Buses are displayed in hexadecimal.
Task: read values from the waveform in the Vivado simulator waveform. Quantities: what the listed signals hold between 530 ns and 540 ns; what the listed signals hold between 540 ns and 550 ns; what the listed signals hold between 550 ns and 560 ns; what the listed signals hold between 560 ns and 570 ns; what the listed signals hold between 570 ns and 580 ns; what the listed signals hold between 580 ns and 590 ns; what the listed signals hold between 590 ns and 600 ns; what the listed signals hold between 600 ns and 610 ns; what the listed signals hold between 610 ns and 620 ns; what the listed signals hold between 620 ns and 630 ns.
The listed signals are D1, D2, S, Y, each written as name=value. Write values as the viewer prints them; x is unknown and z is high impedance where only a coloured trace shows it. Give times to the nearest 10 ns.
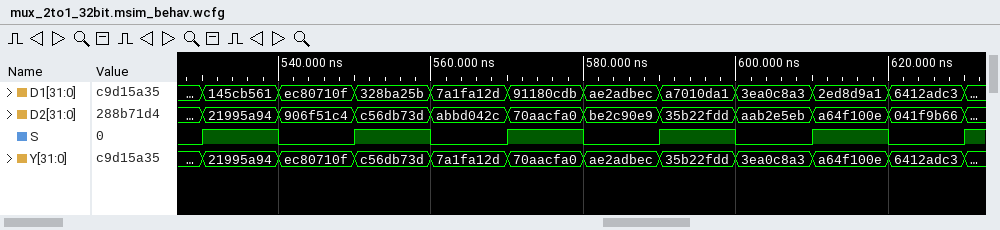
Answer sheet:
D1=145cb561, D2=21995a94, S=1, Y=21995a94
D1=ec80710f, D2=906f51c4, S=0, Y=ec80710f
D1=328ba25b, D2=c56db73d, S=1, Y=c56db73d
D1=7a1fa12d, D2=abbd042c, S=0, Y=7a1fa12d
D1=91180cdb, D2=70aacfa0, S=1, Y=70aacfa0
D1=ae2adbec, D2=be2c90e9, S=0, Y=ae2adbec
D1=a7010da1, D2=35b22fdd, S=1, Y=35b22fdd
D1=3ea0c8a3, D2=aab2e5eb, S=0, Y=3ea0c8a3
D1=2ed8d9a1, D2=a64f100e, S=1, Y=a64f100e
D1=6412adc3, D2=041f9b66, S=0, Y=6412adc3
